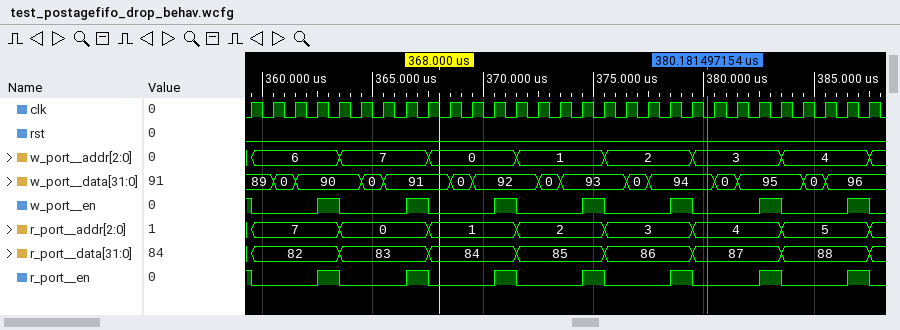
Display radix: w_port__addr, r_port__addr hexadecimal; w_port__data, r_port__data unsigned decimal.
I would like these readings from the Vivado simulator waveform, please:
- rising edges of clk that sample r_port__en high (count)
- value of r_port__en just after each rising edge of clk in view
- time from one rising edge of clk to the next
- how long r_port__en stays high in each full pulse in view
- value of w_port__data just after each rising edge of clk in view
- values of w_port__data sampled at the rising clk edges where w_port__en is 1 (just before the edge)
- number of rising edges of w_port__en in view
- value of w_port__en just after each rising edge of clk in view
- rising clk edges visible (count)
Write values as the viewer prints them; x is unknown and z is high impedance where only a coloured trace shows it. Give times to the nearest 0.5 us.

8
0 0 0 1 0 0 0 1 0 0 0 1 0 0 0 1 0 0 0 1 0 0 0 1 0 0 0 1 0
1 us
1 us, 1 us, 1 us, 1 us, 1 us, 1 us, 1 us
89, 0, 90, 90, 90, 0, 91, 91, 91, 0, 92, 92, 92, 0, 93, 93, 93, 0, 94, 94, 94, 0, 95, 95, 95, 0, 96, 96, 96
89, 90, 91, 92, 93, 94, 95, 96
7
0 0 0 1 0 0 0 1 0 0 0 1 0 0 0 1 0 0 0 1 0 0 0 1 0 0 0 1 0
29
